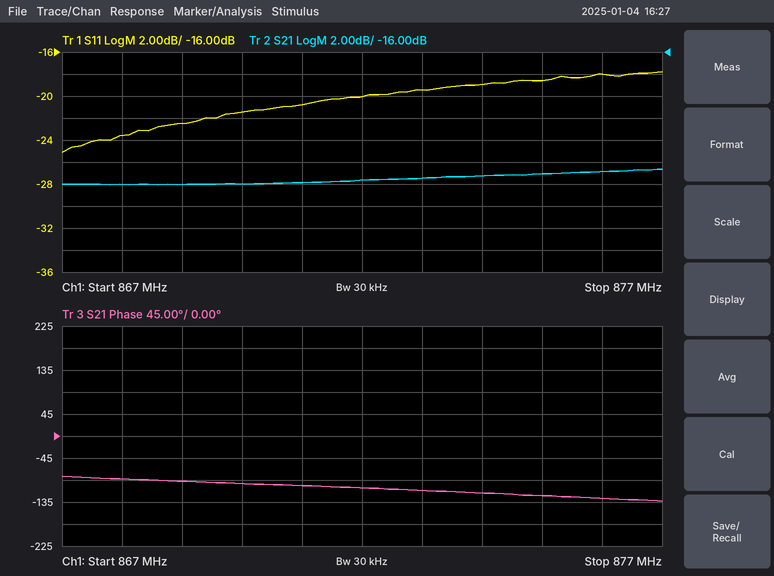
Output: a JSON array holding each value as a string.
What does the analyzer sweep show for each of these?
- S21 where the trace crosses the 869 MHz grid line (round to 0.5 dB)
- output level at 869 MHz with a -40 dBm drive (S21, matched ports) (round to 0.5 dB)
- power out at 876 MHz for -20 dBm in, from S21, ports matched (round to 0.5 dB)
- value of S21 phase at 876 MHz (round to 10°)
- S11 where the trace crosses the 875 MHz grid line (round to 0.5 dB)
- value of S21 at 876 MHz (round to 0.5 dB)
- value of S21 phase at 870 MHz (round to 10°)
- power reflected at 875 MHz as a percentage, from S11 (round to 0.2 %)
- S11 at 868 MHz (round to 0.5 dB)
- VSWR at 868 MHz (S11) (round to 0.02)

["-28.0 dB", "-68.0 dBm", "-47.0 dBm", "-130°", "-18.5 dB", "-27.0 dB", "-100°", "1.4 %", "-23.5 dB", "1.14"]
